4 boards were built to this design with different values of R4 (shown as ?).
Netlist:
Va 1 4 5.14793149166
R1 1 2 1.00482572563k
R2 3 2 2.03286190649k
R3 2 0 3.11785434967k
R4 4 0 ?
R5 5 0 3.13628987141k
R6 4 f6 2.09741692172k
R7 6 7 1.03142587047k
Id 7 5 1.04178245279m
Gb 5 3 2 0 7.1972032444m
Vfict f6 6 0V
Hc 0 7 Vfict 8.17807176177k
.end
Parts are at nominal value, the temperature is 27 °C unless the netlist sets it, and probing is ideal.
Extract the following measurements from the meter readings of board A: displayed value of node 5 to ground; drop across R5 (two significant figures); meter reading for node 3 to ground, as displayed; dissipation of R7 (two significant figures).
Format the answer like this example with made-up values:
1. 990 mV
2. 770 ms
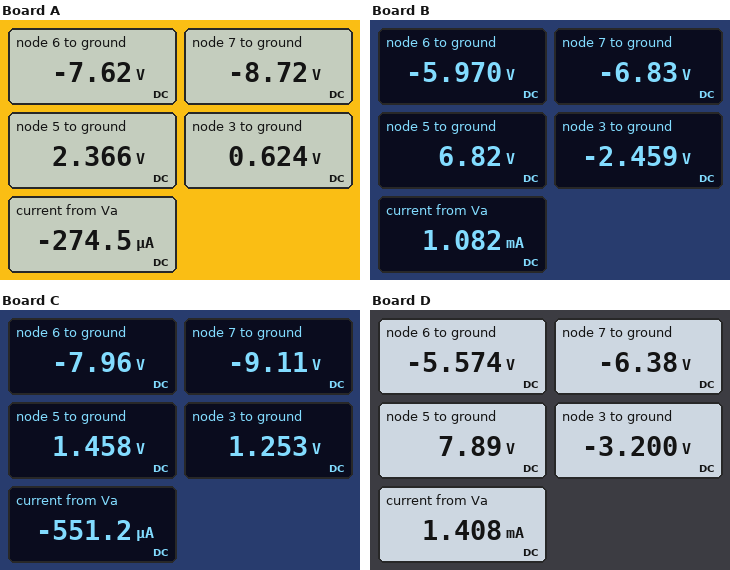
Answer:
1. 2.366 V
2. 2.4 V
3. 0.624 V
4. 1.2 mW
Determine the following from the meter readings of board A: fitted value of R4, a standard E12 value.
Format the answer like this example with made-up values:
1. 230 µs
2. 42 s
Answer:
1. 6.8 kΩ
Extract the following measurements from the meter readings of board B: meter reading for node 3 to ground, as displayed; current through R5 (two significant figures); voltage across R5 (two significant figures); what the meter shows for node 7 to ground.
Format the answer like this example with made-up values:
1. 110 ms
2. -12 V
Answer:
1. -2.459 V
2. 2.2 mA
3. 6.8 V
4. -6.83 V
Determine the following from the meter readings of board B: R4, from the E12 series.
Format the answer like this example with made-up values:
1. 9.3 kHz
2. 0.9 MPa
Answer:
1. 2.2 kΩ
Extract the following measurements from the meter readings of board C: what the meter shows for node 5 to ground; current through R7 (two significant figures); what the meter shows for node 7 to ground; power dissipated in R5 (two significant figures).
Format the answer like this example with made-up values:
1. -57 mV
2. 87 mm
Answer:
1. 1.458 V
2. 1.1 mA
3. -9.11 V
4. 680 µW
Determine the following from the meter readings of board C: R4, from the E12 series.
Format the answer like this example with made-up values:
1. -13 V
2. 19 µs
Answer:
1. 10 kΩ
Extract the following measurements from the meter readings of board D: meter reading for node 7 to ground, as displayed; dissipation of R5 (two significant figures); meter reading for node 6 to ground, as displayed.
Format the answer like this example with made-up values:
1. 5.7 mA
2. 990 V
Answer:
1. -6.38 V
2. 20 mW
3. -5.574 V
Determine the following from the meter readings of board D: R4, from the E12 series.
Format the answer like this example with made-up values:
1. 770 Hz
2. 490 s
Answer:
1. 1.8 kΩ
